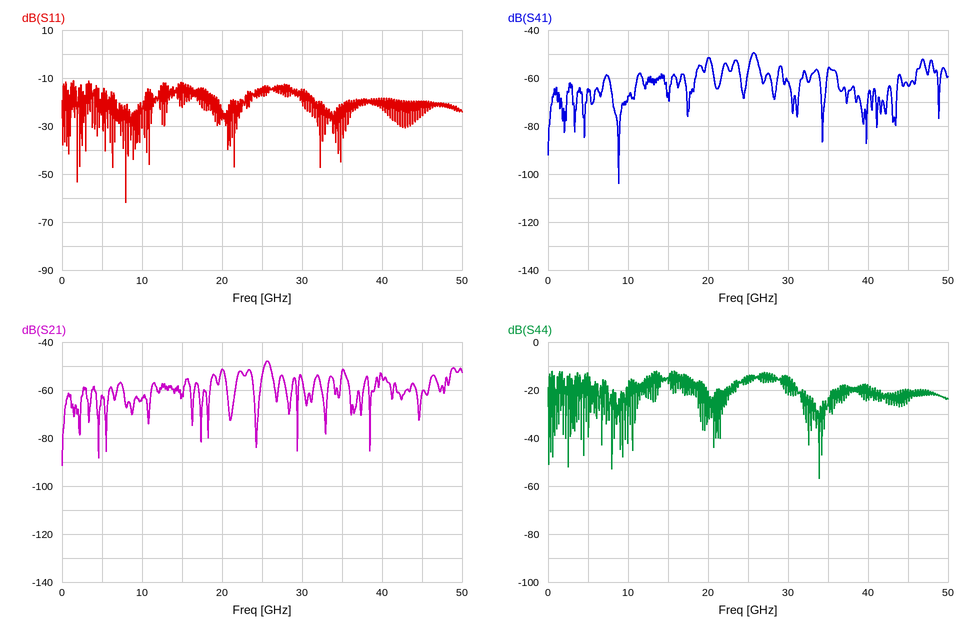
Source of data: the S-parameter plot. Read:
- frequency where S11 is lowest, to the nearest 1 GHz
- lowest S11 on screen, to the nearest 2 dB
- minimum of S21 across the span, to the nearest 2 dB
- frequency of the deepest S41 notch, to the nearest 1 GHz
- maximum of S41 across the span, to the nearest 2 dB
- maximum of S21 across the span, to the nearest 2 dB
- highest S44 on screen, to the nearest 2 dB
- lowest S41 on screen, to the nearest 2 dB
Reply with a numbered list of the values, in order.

1. 8 GHz
2. -62 dB
3. -92 dB
4. 9 GHz
5. -50 dB
6. -48 dB
7. -12 dB
8. -104 dB
